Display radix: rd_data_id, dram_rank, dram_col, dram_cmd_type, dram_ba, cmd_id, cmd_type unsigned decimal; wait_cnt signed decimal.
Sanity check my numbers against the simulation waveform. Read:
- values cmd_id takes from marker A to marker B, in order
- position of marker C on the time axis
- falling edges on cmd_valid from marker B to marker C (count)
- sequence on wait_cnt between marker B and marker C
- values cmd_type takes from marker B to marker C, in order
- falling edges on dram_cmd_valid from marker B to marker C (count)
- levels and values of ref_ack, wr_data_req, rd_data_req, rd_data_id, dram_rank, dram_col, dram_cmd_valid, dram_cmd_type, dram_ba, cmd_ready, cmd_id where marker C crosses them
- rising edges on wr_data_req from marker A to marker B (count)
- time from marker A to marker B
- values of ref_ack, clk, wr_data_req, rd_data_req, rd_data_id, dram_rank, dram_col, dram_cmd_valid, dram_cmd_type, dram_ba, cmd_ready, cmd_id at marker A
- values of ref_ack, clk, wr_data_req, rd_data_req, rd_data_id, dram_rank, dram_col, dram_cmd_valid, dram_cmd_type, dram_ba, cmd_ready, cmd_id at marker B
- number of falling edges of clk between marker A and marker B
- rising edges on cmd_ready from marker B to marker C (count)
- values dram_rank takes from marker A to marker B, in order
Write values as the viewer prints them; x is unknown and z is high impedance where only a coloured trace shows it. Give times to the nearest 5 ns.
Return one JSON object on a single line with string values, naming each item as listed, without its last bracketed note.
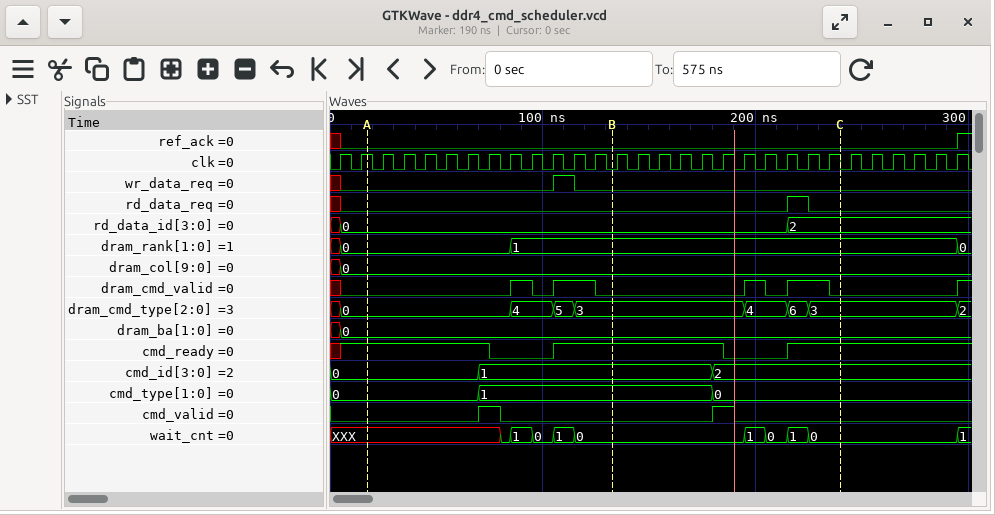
{"values cmd_id takes from marker A to marker B, in order": "0, 1", "position of marker C on the time axis": "240 ns", "falling edges on cmd_valid from marker B to marker C": "1", "sequence on wait_cnt between marker B and marker C": "0, 1, 0, 1, 0", "values cmd_type takes from marker B to marker C, in order": "1, 0", "falling edges on dram_cmd_valid from marker B to marker C": "2", "levels and values of ref_ack, wr_data_req, rd_data_req, rd_data_id, dram_rank, dram_col, dram_cmd_valid, dram_cmd_type, dram_ba, cmd_ready, cmd_id where marker C crosses them": "ref_ack=0, wr_data_req=0, rd_data_req=0, rd_data_id=2, dram_rank=1, dram_col=0, dram_cmd_valid=0, dram_cmd_type=3, dram_ba=0, cmd_ready=1, cmd_id=2", "rising edges on wr_data_req from marker A to marker B": "1", "time from marker A to marker B": "115 ns", "values of ref_ack, clk, wr_data_req, rd_data_req, rd_data_id, dram_rank, dram_col, dram_cmd_valid, dram_cmd_type, dram_ba, cmd_ready, cmd_id at marker A": "ref_ack=0, clk=1, wr_data_req=0, rd_data_req=0, rd_data_id=0, dram_rank=0, dram_col=0, dram_cmd_valid=0, dram_cmd_type=0, dram_ba=0, cmd_ready=1, cmd_id=0", "values of ref_ack, clk, wr_data_req, rd_data_req, rd_data_id, dram_rank, dram_col, dram_cmd_valid, dram_cmd_type, dram_ba, cmd_ready, cmd_id at marker B": "ref_ack=0, clk=0, wr_data_req=0, rd_data_req=0, rd_data_id=0, dram_rank=1, dram_col=0, dram_cmd_valid=0, dram_cmd_type=3, dram_ba=0, cmd_ready=1, cmd_id=1", "number of falling edges of clk between marker A and marker B": "12", "rising edges on cmd_ready from marker B to marker C": "1", "values dram_rank takes from marker A to marker B, in order": "0, 1"}
